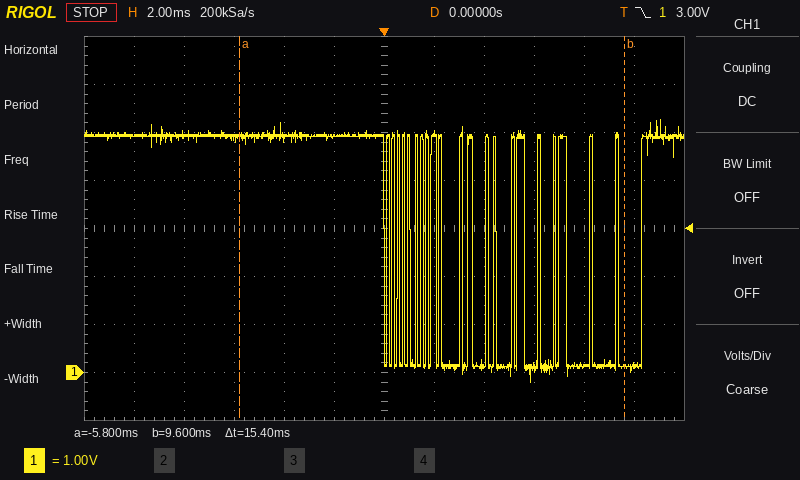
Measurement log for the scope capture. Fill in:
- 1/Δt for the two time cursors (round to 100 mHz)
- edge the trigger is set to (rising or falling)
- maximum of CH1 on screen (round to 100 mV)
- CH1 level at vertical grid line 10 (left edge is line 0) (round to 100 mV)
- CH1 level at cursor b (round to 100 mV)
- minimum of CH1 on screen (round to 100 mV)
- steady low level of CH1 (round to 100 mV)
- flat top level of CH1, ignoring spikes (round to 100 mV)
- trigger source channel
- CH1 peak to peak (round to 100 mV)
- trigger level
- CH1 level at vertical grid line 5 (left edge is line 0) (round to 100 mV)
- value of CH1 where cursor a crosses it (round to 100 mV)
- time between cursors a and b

64.9 Hz
falling
5.3 V
100 mV
100 mV
-200 mV
100 mV
4.9 V
CH1
5.5 V
3.00 V
4.9 V
4.9 V
15.4 ms
